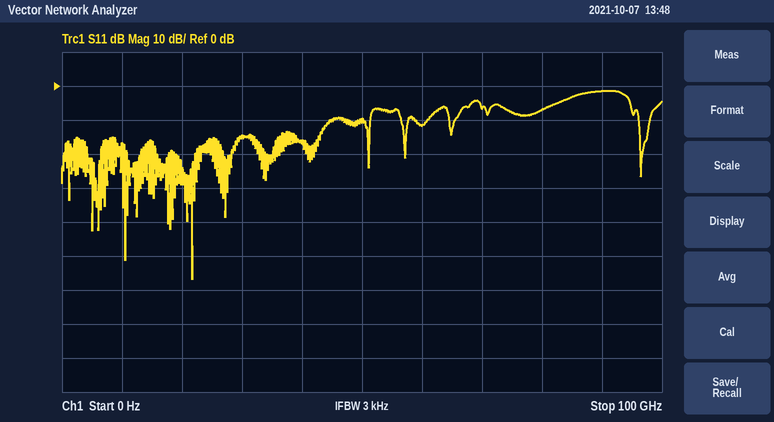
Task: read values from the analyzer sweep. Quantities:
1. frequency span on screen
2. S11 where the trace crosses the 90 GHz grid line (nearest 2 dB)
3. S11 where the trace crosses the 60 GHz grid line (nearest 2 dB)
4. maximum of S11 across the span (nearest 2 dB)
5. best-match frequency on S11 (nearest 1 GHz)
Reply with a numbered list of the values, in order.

1. 100 GHz
2. -2 dB
3. -12 dB
4. -2 dB
5. 22 GHz
